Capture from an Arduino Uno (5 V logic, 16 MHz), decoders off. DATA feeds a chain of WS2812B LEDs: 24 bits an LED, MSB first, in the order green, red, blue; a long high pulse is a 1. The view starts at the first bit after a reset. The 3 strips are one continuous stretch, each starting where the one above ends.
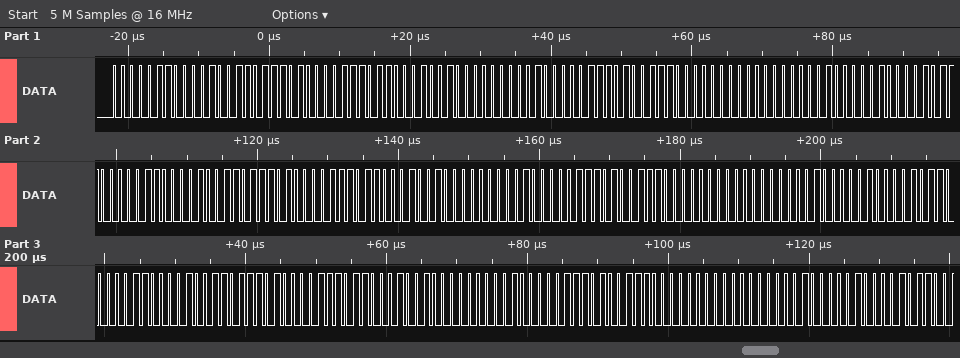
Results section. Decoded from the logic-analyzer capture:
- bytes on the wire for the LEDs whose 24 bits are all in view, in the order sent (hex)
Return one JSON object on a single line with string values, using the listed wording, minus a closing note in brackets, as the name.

{"bytes on the wire for the LEDs whose 24 bits are all in view, in the order sent": "06 13 74 3B 12 00 83 A7 00 00 41 0B 06 13 74 3B 12 00 83 A7 00 00 41 0B 06 13 74 3B 12 00 83 A7 00 00 41 0B"}
